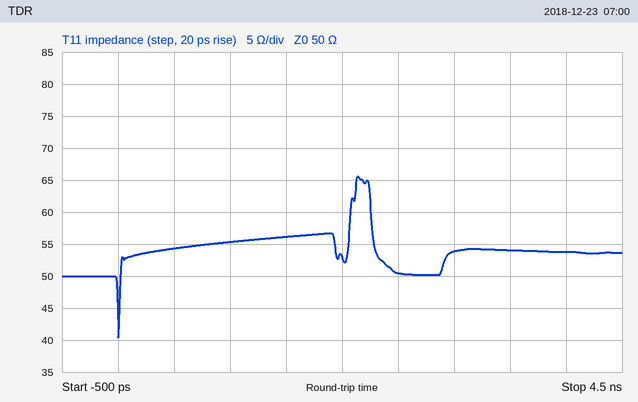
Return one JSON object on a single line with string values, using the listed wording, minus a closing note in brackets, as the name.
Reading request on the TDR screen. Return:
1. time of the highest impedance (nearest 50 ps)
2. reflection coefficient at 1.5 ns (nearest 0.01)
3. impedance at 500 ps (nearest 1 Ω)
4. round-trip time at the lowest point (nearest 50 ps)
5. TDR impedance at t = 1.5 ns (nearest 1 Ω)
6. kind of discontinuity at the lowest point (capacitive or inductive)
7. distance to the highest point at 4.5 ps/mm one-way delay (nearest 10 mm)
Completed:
{"time of the highest impedance": "2.15 ns", "reflection coefficient at 1.5 ns": "+0.06", "impedance at 500 ps": "54 Ω", "round-trip time at the lowest point": "0 ps", "TDR impedance at t = 1.5 ns": "56 Ω", "kind of discontinuity at the lowest point": "capacitive", "distance to the highest point at 4.5 ps/mm one-way delay": "240 mm"}
